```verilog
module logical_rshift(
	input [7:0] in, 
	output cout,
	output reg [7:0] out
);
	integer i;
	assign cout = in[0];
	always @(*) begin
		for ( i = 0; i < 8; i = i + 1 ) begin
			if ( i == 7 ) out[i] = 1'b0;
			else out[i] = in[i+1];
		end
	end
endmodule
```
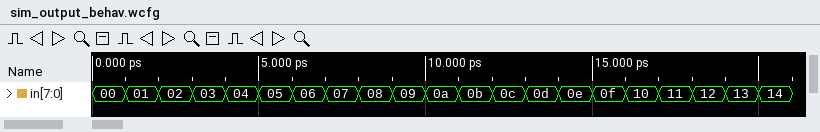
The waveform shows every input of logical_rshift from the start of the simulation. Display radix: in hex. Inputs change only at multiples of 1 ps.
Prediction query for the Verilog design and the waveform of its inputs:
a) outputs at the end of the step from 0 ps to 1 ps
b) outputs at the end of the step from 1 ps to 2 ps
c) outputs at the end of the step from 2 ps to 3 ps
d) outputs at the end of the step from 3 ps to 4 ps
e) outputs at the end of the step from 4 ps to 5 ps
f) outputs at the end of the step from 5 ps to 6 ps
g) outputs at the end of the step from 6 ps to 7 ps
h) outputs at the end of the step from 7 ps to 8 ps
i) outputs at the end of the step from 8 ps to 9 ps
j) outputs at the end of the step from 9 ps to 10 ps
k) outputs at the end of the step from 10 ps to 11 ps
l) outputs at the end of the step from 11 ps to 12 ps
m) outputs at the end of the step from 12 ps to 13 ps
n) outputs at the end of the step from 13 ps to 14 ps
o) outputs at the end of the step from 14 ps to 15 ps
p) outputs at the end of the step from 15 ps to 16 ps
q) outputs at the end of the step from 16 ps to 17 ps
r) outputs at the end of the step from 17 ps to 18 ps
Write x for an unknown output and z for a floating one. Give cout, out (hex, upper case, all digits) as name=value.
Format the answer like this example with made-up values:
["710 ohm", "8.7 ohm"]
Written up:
["cout=0, out=00", "cout=1, out=00", "cout=0, out=01", "cout=1, out=01", "cout=0, out=02", "cout=1, out=02", "cout=0, out=03", "cout=1, out=03", "cout=0, out=04", "cout=1, out=04", "cout=0, out=05", "cout=1, out=05", "cout=0, out=06", "cout=1, out=06", "cout=0, out=07", "cout=1, out=07", "cout=0, out=08", "cout=1, out=08"]
